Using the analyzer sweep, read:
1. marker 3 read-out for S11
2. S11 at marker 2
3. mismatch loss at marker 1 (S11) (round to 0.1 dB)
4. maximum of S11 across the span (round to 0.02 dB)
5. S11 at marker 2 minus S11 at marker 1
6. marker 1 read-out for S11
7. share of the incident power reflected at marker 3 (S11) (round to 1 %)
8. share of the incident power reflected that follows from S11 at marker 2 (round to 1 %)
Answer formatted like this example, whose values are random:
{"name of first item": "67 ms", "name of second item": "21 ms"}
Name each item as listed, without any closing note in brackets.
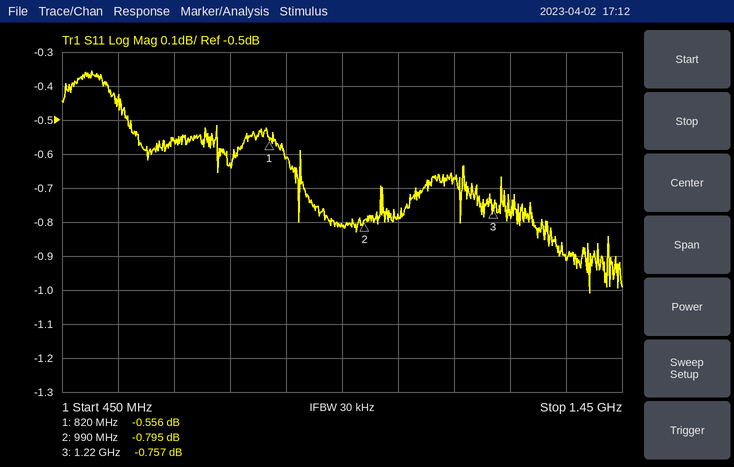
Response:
{"marker 3 read-out for S11": "-0.757 dB", "S11 at marker 2": "-0.795 dB", "mismatch loss at marker 1 (S11)": "9.2 dB", "maximum of S11 across the span": "-0.36 dB", "S11 at marker 2 minus S11 at marker 1": "-0.239 dB", "marker 1 read-out for S11": "-0.556 dB", "share of the incident power reflected at marker 3 (S11)": "84 %", "share of the incident power reflected that follows from S11 at marker 2": "83 %"}
